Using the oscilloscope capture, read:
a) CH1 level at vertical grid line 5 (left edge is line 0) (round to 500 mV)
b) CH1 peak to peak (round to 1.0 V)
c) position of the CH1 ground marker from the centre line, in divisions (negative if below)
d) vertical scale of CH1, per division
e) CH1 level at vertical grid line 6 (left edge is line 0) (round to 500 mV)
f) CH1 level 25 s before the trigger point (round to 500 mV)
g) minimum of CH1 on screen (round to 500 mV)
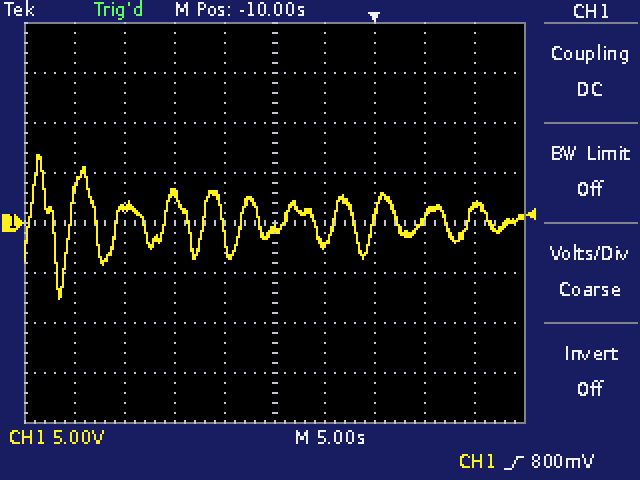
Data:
-500 mV
14.0 V
0.0 div
5 V
-2.0 V
1.5 V
-7.5 V
